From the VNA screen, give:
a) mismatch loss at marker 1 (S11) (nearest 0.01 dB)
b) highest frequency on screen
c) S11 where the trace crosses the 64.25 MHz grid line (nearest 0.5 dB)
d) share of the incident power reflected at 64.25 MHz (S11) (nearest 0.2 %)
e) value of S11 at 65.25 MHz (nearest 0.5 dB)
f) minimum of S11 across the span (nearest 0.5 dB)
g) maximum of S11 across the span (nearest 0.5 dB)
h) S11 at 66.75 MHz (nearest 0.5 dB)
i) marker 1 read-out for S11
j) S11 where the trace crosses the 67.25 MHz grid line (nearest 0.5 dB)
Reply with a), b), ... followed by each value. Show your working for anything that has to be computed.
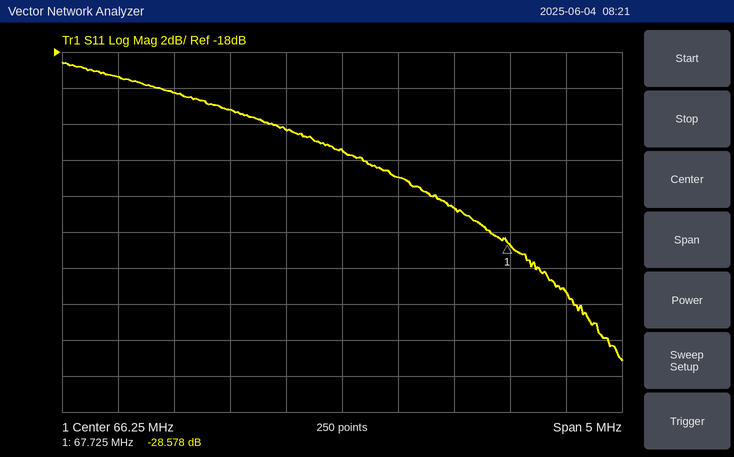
a) −10 log10(1 − 10^(-28.578/10)) ≈ 0.01 dB
b) 68.75 MHz
c) -19.5 dB
d) 10^(-19.5/10) ≈ 1.12 %, so 1.2 % to the nearest 0.2 %
e) -21.0 dB
f) -35.0 dB
g) -18.5 dB
h) -25.0 dB
i) -28.578 dB
j) -26.5 dB
